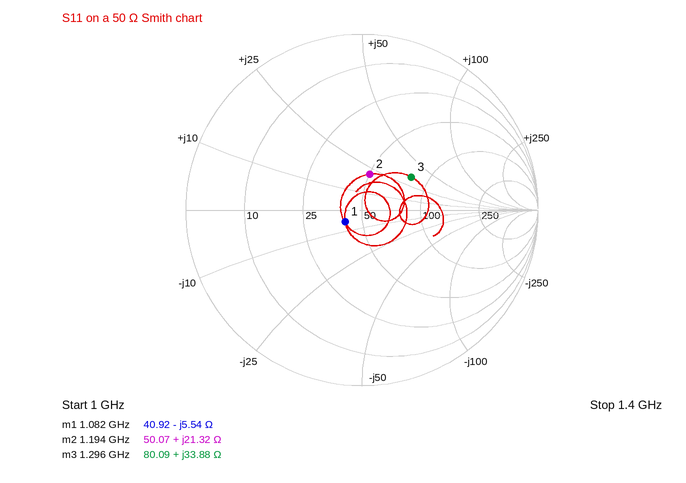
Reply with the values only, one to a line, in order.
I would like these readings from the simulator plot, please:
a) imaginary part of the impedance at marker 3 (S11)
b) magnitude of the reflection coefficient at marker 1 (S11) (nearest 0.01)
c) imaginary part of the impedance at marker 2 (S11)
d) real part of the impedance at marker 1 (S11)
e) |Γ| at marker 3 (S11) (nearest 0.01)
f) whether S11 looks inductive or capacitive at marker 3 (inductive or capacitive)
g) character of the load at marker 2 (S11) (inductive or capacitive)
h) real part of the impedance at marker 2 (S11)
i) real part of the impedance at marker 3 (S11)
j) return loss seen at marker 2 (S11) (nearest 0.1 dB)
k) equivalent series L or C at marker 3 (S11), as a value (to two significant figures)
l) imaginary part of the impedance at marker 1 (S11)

+33.88 Ω
0.12
+21.32 Ω
40.92 Ω
0.34
inductive
inductive
50.07 Ω
80.09 Ω
13.6 dB
4.2 nH
-5.54 Ω
